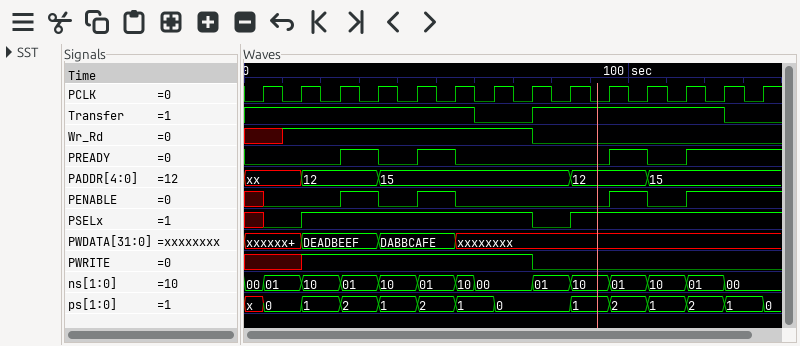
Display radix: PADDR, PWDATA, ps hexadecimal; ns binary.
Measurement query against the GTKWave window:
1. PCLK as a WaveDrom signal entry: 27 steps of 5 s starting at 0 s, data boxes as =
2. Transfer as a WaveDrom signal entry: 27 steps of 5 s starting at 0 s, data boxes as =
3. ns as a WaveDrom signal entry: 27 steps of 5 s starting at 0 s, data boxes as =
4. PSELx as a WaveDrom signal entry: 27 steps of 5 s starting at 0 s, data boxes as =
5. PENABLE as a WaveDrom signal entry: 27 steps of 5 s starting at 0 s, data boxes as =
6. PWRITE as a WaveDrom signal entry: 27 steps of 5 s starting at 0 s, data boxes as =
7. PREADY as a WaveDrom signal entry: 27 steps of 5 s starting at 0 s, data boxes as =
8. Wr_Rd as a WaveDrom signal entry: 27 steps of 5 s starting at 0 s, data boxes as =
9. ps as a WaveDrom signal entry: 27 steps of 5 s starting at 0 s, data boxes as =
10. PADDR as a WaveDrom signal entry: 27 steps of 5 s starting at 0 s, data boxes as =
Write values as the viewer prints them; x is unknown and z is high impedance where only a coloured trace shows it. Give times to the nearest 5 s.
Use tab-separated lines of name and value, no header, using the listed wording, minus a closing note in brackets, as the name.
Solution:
PCLK as a WaveDrom signal entry: 27 steps of 5 s starting at 0 s, data boxes as =	{name: 'PCLK', wave: '010101010101010101010101010'}
Transfer as a WaveDrom signal entry: 27 steps of 5 s starting at 0 s, data boxes as =	{name: 'Transfer', wave: '1...........0..1.........0.'}
ns as a WaveDrom signal entry: 27 steps of 5 s starting at 0 s, data boxes as =	{name: 'ns', wave: '==.=.=.=.=.==..=.=.=.=.=.=.', data: '00 01 10 01 10 01 10 00 01 10 01 10 01 00'}
PSELx as a WaveDrom signal entry: 27 steps of 5 s starting at 0 s, data boxes as =	{name: 'PSELx', wave: 'x0.1...........0.1.........'}
PENABLE as a WaveDrom signal entry: 27 steps of 5 s starting at 0 s, data boxes as =	{name: 'PENABLE', wave: 'x0...1.0.1.0.......1.0.1...'}
PWRITE as a WaveDrom signal entry: 27 steps of 5 s starting at 0 s, data boxes as =	{name: 'PWRITE', wave: 'x..1...........0...........'}
PREADY as a WaveDrom signal entry: 27 steps of 5 s starting at 0 s, data boxes as =	{name: 'PREADY', wave: '0....1.0.1.0.......1.0.1...'}
Wr_Rd as a WaveDrom signal entry: 27 steps of 5 s starting at 0 s, data boxes as =	{name: 'Wr_Rd', wave: 'x.1............0...........'}
ps as a WaveDrom signal entry: 27 steps of 5 s starting at 0 s, data boxes as =	{name: 'ps', wave: 'x=.=.=.=.=.=.=...=.=.=.=.=.', data: '0 1 2 1 2 1 0 1 2 1 2 1'}
PADDR as a WaveDrom signal entry: 27 steps of 5 s starting at 0 s, data boxes as =	{name: 'PADDR', wave: 'x..=...=.........=...=.....', data: '12 15 12 15'}
